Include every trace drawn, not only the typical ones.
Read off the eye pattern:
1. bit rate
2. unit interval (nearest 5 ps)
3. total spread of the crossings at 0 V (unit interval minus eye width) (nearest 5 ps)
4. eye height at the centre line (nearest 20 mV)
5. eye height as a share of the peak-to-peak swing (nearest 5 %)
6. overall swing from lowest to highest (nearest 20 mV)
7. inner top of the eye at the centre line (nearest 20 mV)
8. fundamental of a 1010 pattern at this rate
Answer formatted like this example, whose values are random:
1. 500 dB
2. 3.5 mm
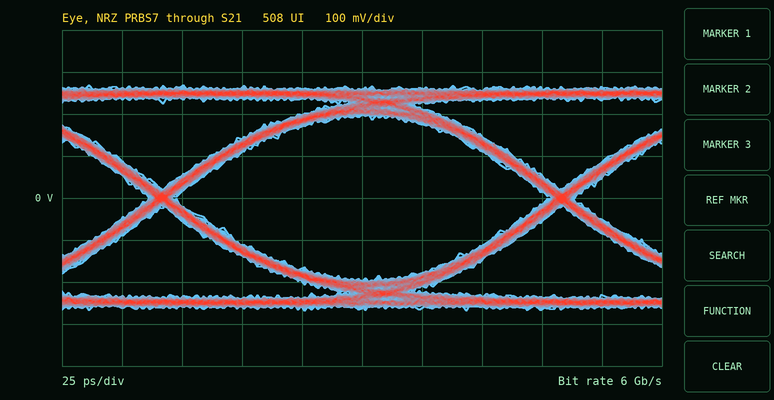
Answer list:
1. 6 Gb/s
2. 165 ps
3. 10 ps
4. 400 mV
5. 75 %
6. 540 mV
7. 200 mV
8. 3 GHz
